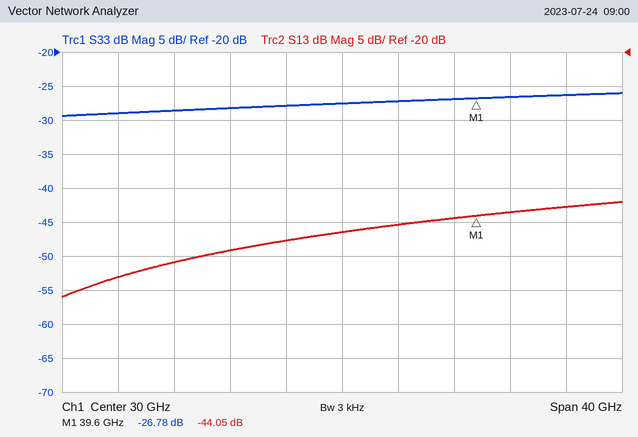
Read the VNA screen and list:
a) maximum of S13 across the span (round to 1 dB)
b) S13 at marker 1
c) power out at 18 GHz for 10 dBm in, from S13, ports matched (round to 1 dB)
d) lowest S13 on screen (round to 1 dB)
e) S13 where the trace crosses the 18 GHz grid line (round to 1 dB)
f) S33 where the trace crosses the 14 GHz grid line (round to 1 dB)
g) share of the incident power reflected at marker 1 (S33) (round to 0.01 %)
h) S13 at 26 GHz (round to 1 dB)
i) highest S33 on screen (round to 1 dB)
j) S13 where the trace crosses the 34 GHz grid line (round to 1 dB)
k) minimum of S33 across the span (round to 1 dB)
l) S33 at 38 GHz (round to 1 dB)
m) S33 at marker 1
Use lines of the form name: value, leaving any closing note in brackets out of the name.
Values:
maximum of S13 across the span: -42 dB
S13 at marker 1: -44.05 dB
power out at 18 GHz for 10 dBm in, from S13, ports matched: -41 dBm
lowest S13 on screen: -56 dB
S13 where the trace crosses the 18 GHz grid line: -51 dB
S33 where the trace crosses the 14 GHz grid line: -29 dB
share of the incident power reflected at marker 1 (S33): 0.21 %
S13 at 26 GHz: -48 dB
highest S33 on screen: -26 dB
S13 where the trace crosses the 34 GHz grid line: -45 dB
minimum of S33 across the span: -29 dB
S33 at 38 GHz: -27 dB
S33 at marker 1: -26.78 dB
